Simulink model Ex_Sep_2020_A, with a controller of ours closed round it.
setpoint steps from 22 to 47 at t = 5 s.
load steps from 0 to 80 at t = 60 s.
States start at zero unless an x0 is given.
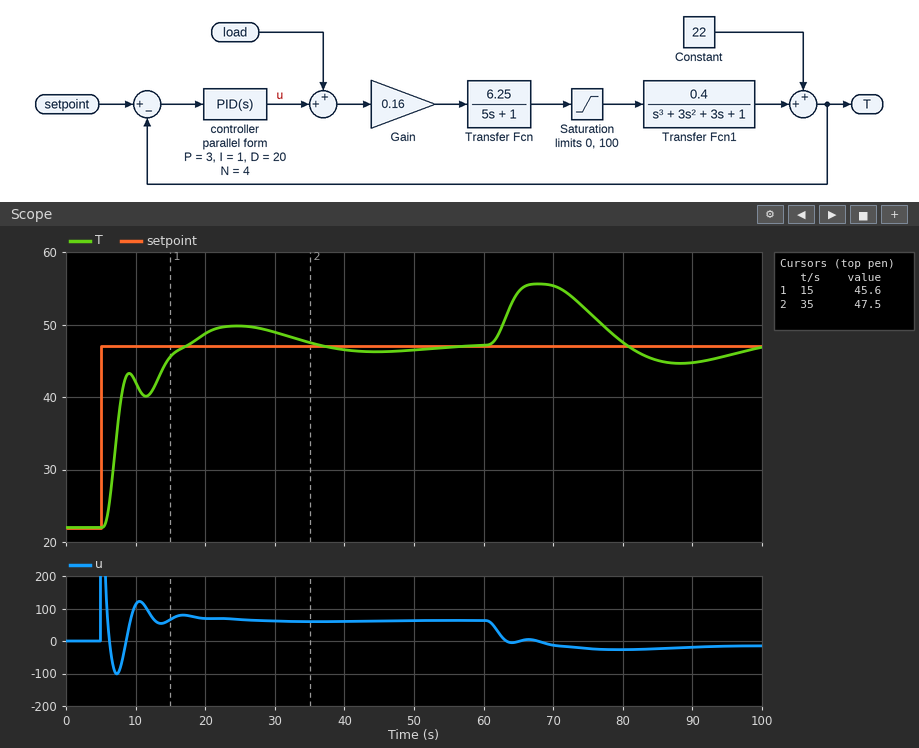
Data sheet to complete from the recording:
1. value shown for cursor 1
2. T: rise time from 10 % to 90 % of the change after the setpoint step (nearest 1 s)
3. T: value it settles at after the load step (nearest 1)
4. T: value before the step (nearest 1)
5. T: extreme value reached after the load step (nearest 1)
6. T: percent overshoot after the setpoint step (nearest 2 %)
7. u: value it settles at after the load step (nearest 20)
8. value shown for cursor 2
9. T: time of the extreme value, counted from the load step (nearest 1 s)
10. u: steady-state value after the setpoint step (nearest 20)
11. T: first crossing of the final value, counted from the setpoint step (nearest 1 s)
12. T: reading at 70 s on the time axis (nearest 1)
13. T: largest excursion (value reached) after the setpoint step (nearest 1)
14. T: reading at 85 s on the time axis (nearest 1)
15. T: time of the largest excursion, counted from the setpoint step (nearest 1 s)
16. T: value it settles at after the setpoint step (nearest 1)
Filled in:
45.6
8 s
47
22
56
12 %
-20
47.5
8 s
60
12 s
55
50
45
20 s
47
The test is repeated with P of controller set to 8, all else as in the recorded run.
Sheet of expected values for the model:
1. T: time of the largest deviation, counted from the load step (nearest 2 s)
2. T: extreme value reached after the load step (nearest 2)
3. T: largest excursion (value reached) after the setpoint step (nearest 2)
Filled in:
6 s
54
50
